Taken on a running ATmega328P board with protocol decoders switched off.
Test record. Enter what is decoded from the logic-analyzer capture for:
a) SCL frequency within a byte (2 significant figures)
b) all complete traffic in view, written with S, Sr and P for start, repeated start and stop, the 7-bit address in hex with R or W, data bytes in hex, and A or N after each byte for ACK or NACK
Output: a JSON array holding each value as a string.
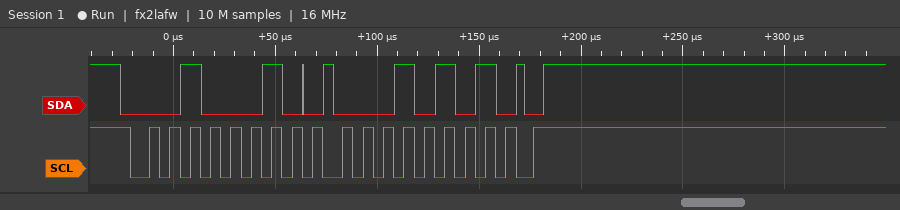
["100 kHz", "S 11W A 15 A P"]
